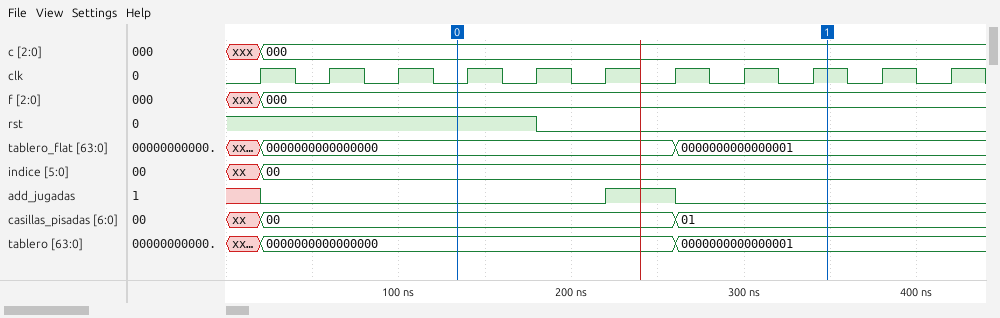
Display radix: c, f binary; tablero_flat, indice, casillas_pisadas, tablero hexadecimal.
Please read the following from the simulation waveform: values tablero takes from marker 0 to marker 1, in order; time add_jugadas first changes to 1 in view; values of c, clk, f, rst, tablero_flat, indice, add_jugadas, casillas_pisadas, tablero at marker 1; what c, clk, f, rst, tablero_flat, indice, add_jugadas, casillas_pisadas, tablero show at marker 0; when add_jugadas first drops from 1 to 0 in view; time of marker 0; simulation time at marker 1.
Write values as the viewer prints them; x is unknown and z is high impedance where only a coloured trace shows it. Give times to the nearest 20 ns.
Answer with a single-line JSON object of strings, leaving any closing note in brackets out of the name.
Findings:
{"values tablero takes from marker 0 to marker 1, in order": "0000000000000000, 0000000000000001", "time add_jugadas first changes to 1 in view": "220 ns", "values of c, clk, f, rst, tablero_flat, indice, add_jugadas, casillas_pisadas, tablero at marker 1": "c=000, clk=1, f=000, rst=0, tablero_flat=0000000000000001, indice=00, add_jugadas=0, casillas_pisadas=01, tablero=0000000000000001", "what c, clk, f, rst, tablero_flat, indice, add_jugadas, casillas_pisadas, tablero show at marker 0": "c=000, clk=0, f=000, rst=1, tablero_flat=0000000000000000, indice=00, add_jugadas=0, casillas_pisadas=00, tablero=0000000000000000", "when add_jugadas first drops from 1 to 0 in view": "260 ns", "time of marker 0": "140 ns", "simulation time at marker 1": "340 ns"}
